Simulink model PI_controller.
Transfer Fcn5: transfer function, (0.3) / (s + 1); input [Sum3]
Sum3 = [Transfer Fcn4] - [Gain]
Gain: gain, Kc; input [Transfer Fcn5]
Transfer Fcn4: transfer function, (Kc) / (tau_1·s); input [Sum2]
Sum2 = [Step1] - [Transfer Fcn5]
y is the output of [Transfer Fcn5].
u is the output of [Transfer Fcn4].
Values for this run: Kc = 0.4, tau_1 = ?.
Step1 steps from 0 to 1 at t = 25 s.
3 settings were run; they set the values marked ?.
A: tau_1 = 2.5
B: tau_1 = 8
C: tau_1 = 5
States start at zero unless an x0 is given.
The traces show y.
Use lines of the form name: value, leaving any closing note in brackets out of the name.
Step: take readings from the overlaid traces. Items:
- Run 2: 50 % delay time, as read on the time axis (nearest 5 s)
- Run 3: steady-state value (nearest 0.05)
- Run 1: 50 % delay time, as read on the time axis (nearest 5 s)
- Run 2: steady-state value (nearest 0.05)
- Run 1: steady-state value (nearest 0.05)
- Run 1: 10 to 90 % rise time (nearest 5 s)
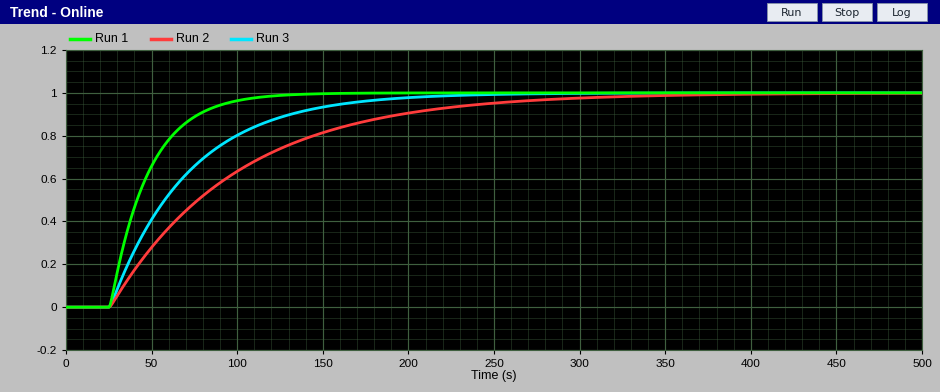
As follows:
Run 2: 50 % delay time, as read on the time axis: 75 s
Run 3: steady-state value: 1.00
Run 1: 50 % delay time, as read on the time axis: 40 s
Run 2: steady-state value: 1.00
Run 1: steady-state value: 1.00
Run 1: 10 to 90 % rise time: 50 s
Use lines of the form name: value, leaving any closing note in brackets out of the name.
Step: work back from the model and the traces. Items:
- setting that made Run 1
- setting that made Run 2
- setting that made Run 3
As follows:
setting that made Run 1: A
setting that made Run 2: B
setting that made Run 3: C
